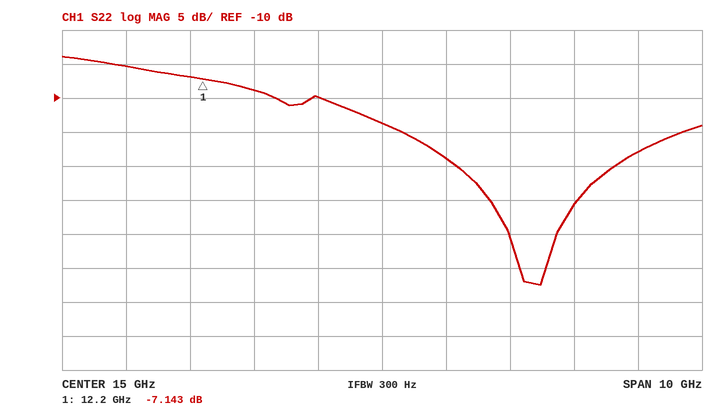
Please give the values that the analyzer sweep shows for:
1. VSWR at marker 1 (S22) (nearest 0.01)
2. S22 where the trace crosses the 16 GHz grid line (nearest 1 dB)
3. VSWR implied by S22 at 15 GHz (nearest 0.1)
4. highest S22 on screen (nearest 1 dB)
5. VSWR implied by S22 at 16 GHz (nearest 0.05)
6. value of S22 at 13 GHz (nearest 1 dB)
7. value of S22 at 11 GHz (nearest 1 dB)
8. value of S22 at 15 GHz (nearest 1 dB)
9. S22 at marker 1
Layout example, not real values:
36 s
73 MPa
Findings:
2.57
-19 dB
1.5
-4 dB
1.25
-9 dB
-5 dB
-14 dB
-7.143 dB
